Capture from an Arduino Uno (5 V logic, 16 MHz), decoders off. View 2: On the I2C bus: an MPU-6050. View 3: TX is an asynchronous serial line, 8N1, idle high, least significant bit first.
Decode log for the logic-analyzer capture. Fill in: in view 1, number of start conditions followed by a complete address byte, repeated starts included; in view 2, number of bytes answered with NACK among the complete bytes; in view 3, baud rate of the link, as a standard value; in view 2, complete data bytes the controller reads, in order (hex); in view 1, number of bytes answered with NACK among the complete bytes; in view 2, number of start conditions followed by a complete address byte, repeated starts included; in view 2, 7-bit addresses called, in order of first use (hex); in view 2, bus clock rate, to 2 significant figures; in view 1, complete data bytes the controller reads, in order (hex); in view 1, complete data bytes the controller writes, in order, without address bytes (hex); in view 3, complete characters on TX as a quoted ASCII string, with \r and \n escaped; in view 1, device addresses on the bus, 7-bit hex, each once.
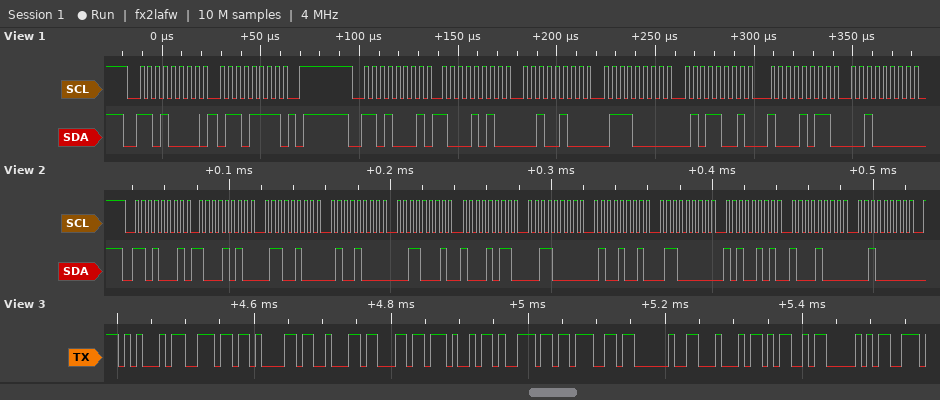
2
0
115200 baud
8A 64 48 31 8B 30 49 60 A5 88 20
0
1
0x68
250 kHz
8A 24 70 59 8B 20
6F
"Enabling DMP"
0x68
